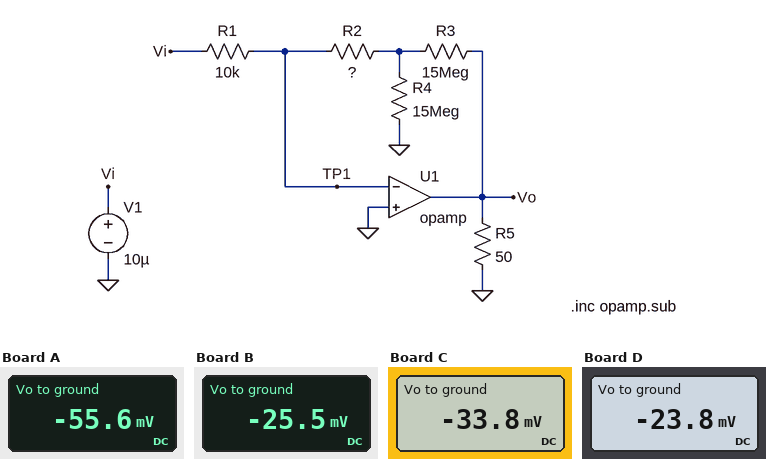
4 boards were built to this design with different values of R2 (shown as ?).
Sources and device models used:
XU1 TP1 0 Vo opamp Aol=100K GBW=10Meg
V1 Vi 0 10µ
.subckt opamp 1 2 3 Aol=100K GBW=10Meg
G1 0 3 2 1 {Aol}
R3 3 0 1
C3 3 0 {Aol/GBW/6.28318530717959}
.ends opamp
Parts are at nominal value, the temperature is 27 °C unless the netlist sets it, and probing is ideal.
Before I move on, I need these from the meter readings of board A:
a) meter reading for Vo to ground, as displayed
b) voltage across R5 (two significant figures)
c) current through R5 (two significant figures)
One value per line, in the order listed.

-55.6 mV
56 mV
1.1 mA
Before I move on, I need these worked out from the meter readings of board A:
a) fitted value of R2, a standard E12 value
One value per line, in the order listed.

22 MΩ
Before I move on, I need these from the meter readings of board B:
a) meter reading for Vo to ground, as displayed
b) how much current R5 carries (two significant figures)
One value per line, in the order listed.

-25.5 mV
510 µA
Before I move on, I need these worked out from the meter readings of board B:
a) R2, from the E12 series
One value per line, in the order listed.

5.6 MΩ
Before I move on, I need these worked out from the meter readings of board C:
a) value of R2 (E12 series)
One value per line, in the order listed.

10 MΩ
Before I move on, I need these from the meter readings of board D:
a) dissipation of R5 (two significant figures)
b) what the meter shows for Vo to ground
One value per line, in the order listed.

11 µW
-23.8 mV
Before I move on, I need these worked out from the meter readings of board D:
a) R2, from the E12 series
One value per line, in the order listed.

4.7 MΩ
